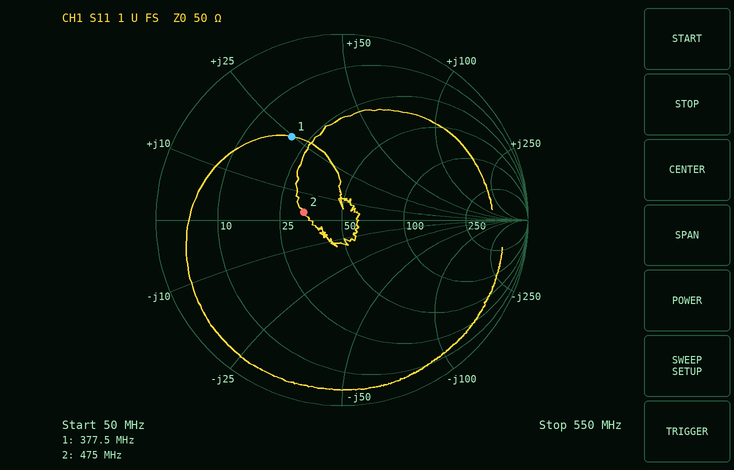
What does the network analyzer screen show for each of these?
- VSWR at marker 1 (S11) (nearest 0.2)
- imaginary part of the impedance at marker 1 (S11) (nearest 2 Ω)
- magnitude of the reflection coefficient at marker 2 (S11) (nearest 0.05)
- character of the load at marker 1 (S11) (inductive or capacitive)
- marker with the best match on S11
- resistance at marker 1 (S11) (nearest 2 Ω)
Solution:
3.2
+24 Ω
0.20
inductive
marker 2
20 Ω
